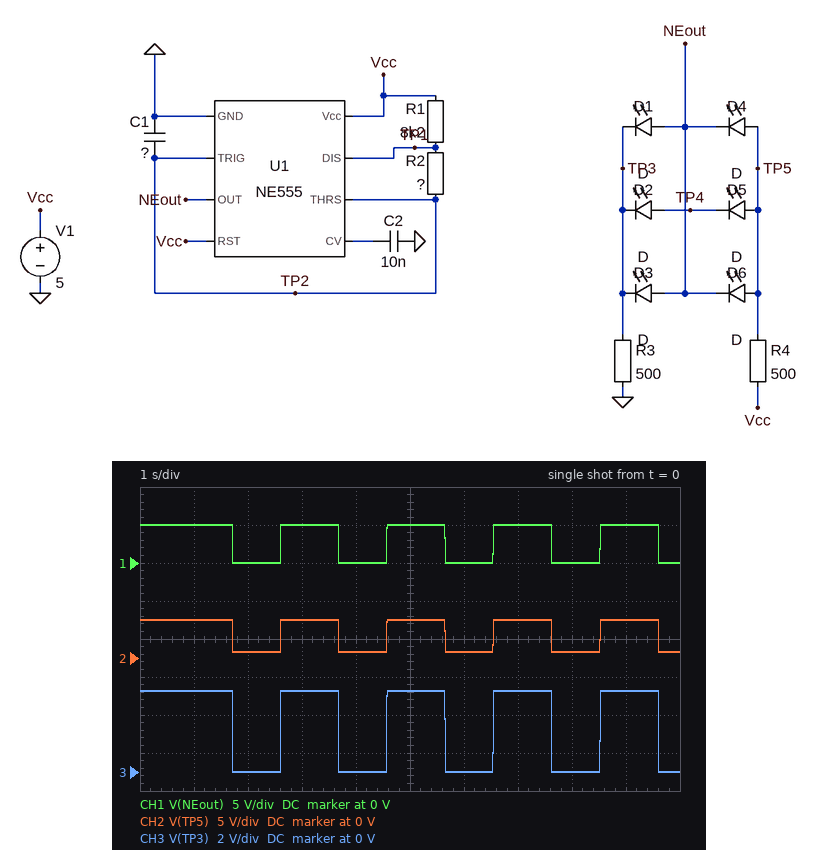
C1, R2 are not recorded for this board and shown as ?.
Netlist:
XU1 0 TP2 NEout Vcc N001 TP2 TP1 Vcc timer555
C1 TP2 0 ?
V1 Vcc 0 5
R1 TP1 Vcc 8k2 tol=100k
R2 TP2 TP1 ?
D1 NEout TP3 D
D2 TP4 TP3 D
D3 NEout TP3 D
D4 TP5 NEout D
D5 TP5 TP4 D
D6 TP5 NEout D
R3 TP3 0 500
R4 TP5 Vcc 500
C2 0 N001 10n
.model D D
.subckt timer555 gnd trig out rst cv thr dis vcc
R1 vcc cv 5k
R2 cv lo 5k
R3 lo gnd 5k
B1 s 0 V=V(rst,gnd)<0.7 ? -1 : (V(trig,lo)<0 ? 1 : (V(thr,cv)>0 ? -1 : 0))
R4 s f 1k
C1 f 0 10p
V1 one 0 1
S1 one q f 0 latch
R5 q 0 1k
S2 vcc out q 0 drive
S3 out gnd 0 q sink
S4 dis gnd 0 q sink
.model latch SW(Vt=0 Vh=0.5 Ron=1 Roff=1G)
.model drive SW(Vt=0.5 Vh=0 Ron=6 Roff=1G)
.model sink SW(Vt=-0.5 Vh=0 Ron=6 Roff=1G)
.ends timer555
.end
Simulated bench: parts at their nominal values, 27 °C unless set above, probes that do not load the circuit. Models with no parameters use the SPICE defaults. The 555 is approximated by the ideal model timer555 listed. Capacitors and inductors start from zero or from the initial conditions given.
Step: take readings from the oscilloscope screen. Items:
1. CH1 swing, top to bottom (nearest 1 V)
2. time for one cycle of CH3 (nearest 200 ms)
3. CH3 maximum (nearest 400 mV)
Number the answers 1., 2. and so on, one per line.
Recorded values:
1. 5 V
2. 2.0 s
3. 4.4 V
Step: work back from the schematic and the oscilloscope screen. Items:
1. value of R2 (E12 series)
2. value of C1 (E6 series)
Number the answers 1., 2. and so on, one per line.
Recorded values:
1. 39 kΩ
2. 33 µF
